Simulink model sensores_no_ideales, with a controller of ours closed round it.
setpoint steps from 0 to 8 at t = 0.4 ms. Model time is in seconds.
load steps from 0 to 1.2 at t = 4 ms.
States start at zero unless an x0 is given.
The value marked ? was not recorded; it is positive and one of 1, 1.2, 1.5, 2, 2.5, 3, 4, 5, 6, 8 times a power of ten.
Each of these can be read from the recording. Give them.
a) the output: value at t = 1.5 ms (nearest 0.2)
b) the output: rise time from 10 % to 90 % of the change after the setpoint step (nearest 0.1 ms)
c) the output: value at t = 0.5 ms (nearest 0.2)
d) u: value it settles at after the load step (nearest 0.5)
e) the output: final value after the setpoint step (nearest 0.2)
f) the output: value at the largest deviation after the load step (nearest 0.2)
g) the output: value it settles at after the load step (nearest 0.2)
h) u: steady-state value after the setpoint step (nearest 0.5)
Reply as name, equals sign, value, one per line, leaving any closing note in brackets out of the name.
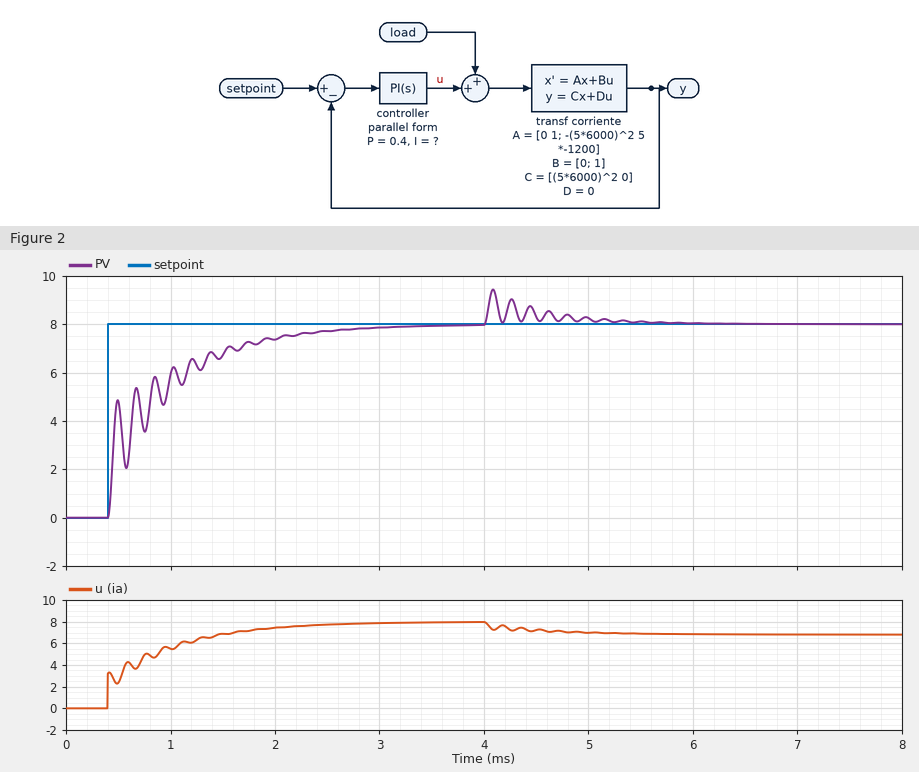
the output: value at t = 1.5 ms = 6.8
the output: rise time from 10 % to 90 % of the change after the setpoint step = 1.3 ms
the output: value at t = 0.5 ms = 4.8
u: value it settles at after the load step = 7.0
the output: final value after the setpoint step = 8.0
the output: value at the largest deviation after the load step = 9.4
the output: value it settles at after the load step = 8.0
u: steady-state value after the setpoint step = 8.0
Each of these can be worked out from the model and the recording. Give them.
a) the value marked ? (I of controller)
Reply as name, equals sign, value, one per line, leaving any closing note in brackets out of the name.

the value marked ? = 2000
